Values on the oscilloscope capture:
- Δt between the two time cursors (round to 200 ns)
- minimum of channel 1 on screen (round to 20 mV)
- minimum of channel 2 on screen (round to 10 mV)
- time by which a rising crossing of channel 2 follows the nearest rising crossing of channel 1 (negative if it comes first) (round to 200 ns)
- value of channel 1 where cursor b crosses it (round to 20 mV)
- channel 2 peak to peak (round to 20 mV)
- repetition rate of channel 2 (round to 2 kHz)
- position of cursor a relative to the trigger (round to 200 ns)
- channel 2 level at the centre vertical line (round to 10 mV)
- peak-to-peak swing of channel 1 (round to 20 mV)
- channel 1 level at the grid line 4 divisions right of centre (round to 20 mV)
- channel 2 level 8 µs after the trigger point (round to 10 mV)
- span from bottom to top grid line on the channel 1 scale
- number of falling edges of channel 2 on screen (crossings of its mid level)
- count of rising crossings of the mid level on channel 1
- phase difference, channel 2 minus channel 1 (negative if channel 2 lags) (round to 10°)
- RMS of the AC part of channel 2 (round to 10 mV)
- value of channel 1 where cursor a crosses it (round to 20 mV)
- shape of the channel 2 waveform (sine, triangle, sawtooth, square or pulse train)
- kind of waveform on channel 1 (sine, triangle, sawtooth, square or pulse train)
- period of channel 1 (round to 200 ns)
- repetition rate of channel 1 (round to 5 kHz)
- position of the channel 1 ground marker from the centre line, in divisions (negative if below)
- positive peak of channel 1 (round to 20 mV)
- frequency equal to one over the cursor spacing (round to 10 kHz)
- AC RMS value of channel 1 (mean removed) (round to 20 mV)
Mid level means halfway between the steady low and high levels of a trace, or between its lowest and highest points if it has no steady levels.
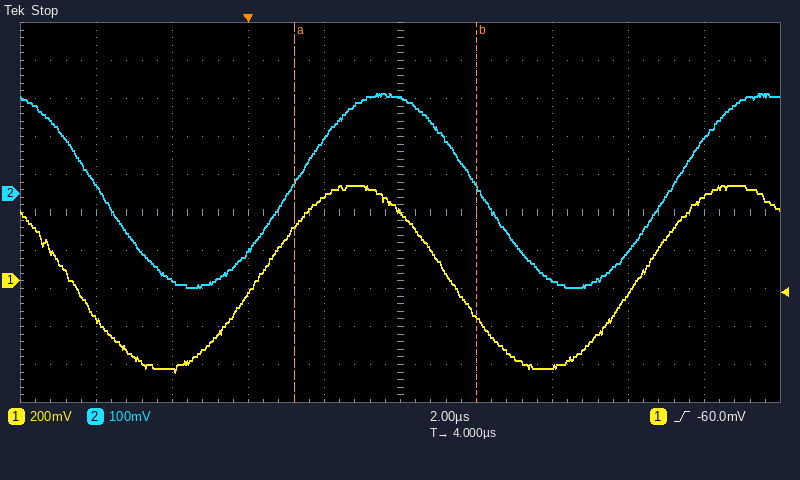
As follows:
4.8 µs
-480 mV
-250 mV
+800 ns
-200 mV
520 mV
100 kHz
+1.2 µs
250 mV
980 mV
440 mV
-230 mV
2 V
2
2
-30°
180 mV
280 mV
sine
sine
10.0 µs
100 kHz
-1.8 div
500 mV
210 kHz
340 mV
